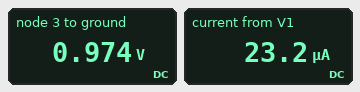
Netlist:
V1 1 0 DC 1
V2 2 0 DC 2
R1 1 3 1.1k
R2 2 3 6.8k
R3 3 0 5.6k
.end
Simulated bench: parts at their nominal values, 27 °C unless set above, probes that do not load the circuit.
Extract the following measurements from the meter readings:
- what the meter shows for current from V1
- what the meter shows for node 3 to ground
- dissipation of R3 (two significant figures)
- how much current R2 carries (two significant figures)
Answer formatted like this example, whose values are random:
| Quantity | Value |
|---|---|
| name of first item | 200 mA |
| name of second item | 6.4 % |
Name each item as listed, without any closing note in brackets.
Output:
| Quantity | Value |
|---|---|
| what the meter shows for current from V1 | 23.2 µA |
| what the meter shows for node 3 to ground | 0.974 V |
| dissipation of R3 | 170 µW |
| how much current R2 carries | 150 µA |
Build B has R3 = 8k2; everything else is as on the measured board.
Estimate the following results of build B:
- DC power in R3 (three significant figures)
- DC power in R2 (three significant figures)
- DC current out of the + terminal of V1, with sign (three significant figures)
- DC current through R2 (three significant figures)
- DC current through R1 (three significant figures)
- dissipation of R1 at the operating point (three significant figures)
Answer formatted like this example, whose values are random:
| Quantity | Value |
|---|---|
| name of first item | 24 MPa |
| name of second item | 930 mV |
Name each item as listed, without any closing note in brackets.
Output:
| Quantity | Value |
|---|---|
| DC power in R3 | 127 µW |
| DC power in R2 | 141 µW |
| DC current out of the + terminal of V1, with sign | -19.4 µA |
| DC current through R2 | 144 µA |
| DC current through R1 | 19.4 µA |
| dissipation of R1 at the operating point | 413 nW |
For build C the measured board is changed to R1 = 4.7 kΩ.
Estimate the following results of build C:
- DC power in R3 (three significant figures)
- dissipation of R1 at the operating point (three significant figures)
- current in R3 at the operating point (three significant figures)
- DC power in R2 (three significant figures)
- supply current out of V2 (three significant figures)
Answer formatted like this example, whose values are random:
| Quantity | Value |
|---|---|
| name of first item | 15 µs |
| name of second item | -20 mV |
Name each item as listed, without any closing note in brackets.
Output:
| Quantity | Value |
|---|---|
| DC power in R3 | 158 µW |
| dissipation of R1 at the operating point | 729 nW |
| current in R3 at the operating point | 168 µA |
| DC power in R2 | 165 µW |
| supply current out of V2 | 156 µA |
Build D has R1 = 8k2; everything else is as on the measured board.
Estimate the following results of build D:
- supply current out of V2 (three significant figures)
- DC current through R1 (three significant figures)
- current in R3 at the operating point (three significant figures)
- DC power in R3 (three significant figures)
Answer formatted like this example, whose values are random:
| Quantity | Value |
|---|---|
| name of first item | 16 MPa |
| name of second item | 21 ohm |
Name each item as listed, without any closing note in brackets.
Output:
| Quantity | Value |
|---|---|
| supply current out of V2 | 157 µA |
| DC current through R1 | 8.59 µA |
| current in R3 at the operating point | 166 µA |
| DC power in R3 | 154 µW |
